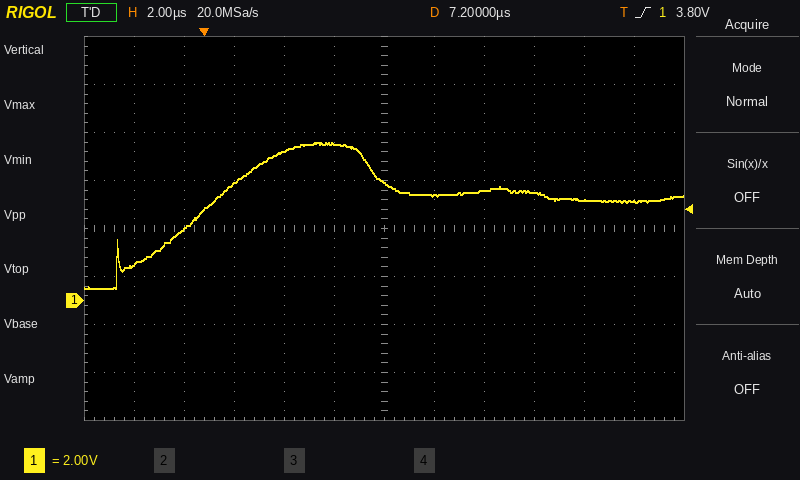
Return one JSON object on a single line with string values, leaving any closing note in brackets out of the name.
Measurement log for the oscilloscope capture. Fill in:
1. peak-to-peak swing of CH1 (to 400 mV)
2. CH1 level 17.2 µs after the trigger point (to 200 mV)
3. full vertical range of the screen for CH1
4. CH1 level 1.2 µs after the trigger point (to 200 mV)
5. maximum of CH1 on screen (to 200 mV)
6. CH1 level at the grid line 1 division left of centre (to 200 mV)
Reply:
{"peak-to-peak swing of CH1": "6.0 V", "CH1 level 17.2 µs after the trigger point": "4.2 V", "full vertical range of the screen for CH1": "16 V", "CH1 level 1.2 µs after the trigger point": "4.8 V", "maximum of CH1 on screen": "6.6 V", "CH1 level at the grid line 1 division left of centre": "6.6 V"}
